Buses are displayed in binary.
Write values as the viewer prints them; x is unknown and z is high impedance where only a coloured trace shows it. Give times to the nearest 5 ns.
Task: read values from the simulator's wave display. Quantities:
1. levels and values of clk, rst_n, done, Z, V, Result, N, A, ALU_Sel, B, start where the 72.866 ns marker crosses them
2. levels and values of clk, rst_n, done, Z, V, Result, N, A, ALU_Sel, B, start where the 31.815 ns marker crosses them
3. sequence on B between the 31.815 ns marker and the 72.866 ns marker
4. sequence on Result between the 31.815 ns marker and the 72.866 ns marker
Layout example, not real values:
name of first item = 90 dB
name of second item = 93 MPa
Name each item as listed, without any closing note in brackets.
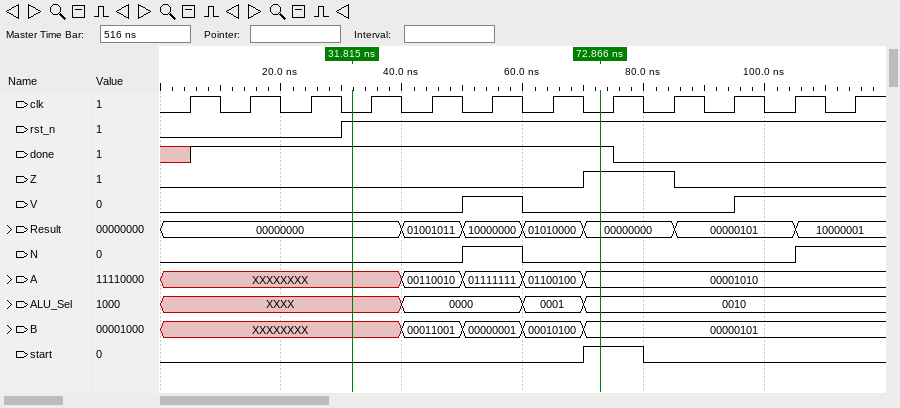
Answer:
levels and values of clk, rst_n, done, Z, V, Result, N, A, ALU_Sel, B, start where the 72.866 ns marker crosses them = clk=0, rst_n=1, done=1, Z=1, V=0, Result=00000000, N=0, A=00001010, ALU_Sel=0010, B=00000101, start=1
levels and values of clk, rst_n, done, Z, V, Result, N, A, ALU_Sel, B, start where the 31.815 ns marker crosses them = clk=0, rst_n=1, done=1, Z=0, V=0, Result=00000000, N=0, A=XXXXXXXX, ALU_Sel=XXXX, B=XXXXXXXX, start=0
sequence on B between the 31.815 ns marker and the 72.866 ns marker = XXXXXXXX, 00011001, 00000001, 00010100, 00000101
sequence on Result between the 31.815 ns marker and the 72.866 ns marker = 00000000, 01001011, 10000000, 01010000, 00000000
